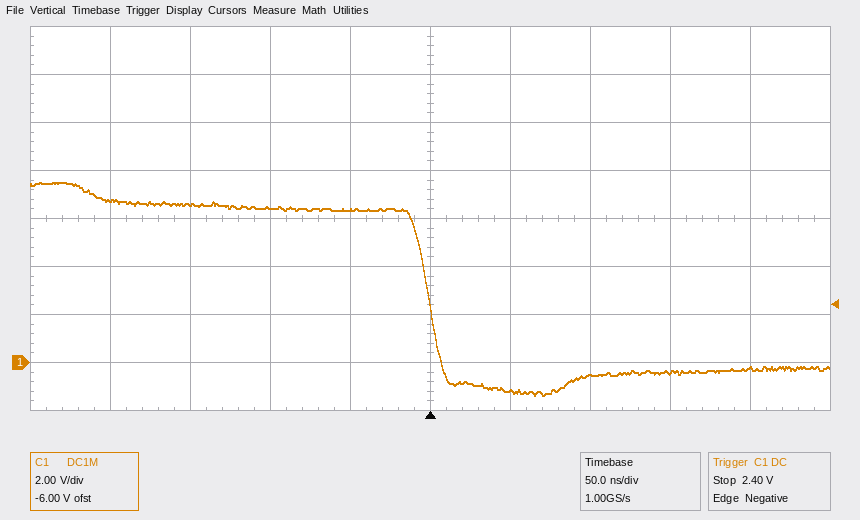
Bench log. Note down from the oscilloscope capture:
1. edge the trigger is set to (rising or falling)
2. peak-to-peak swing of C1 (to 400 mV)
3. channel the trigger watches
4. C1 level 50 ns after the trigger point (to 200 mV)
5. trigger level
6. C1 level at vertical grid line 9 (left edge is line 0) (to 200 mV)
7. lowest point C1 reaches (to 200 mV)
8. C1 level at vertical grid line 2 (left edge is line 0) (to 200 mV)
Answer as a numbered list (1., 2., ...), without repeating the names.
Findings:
1. falling
2. 8.8 V
3. C1
4. -1.2 V
5. 2.40 V
6. -200 mV
7. -1.4 V
8. 6.6 V
